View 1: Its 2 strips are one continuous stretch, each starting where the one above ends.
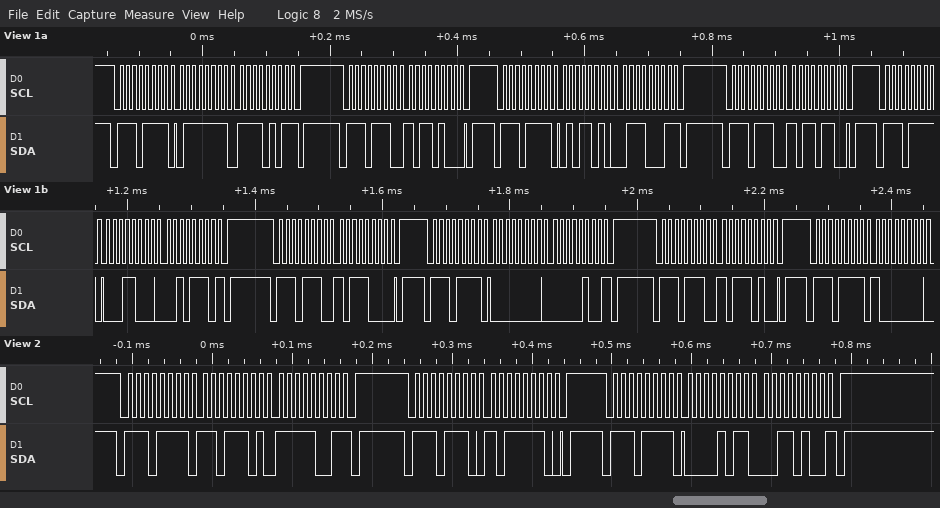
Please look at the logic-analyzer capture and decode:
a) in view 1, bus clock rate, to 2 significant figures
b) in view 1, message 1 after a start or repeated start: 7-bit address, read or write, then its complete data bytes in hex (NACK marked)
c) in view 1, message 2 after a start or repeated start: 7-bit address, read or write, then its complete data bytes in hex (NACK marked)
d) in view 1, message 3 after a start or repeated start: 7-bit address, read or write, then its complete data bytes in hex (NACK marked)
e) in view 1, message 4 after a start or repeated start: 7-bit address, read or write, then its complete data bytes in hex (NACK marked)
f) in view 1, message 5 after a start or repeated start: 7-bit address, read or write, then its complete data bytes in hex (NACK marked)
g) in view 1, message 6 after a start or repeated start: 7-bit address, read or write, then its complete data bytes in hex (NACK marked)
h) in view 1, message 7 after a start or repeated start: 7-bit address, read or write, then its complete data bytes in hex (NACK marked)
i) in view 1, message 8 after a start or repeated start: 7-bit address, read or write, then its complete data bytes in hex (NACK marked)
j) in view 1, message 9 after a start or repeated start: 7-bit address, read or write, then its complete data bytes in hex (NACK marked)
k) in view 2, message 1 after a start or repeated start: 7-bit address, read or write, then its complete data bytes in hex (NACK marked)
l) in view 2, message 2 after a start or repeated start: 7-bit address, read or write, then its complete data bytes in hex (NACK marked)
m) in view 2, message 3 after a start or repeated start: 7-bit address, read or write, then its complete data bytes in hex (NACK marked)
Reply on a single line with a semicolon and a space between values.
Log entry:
100 kHz; 0x77 read: 7F F5 NACK; 0x77 write: B4; 0x77 read: 5A 71 NACK; 0x77 write: B6; 0x77 read: 18 2E NACK; 0x77 write: B8; 0x77 read: 00 04 NACK; 0x77 write: BA; 0x77 read: 80; 0x77 read: DD F9 NACK; 0x77 write: BE; 0x77 read: 0B 34 NACK
